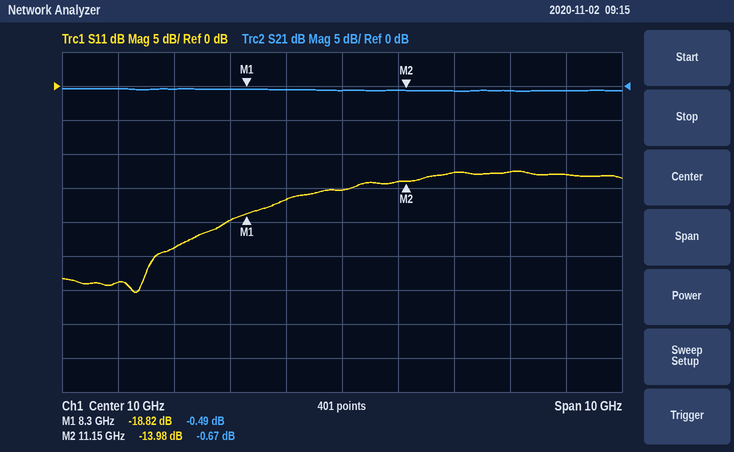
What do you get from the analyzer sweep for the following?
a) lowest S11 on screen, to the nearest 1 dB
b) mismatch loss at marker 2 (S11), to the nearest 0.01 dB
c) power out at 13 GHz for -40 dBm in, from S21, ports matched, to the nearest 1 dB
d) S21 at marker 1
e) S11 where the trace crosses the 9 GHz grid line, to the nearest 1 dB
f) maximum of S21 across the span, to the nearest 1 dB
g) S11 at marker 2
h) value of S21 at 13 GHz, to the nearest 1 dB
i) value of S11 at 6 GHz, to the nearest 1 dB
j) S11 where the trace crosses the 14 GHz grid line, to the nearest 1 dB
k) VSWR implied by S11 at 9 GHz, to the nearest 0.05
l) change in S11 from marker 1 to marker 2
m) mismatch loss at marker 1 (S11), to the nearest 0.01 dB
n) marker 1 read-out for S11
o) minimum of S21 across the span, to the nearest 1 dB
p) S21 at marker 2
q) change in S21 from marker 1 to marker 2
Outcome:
-30 dB
0.18 dB
-41 dBm
-0.49 dB
-17 dB
0 dB
-13.98 dB
-1 dB
-29 dB
-13 dB
1.35
4.84 dB
0.06 dB
-18.82 dB
-1 dB
-0.67 dB
-0.18 dB
